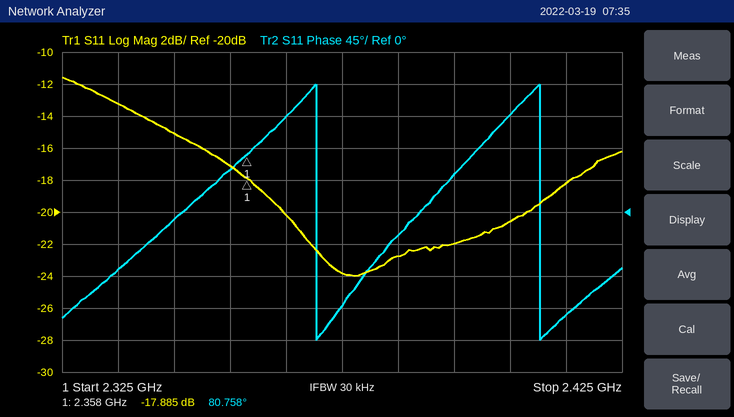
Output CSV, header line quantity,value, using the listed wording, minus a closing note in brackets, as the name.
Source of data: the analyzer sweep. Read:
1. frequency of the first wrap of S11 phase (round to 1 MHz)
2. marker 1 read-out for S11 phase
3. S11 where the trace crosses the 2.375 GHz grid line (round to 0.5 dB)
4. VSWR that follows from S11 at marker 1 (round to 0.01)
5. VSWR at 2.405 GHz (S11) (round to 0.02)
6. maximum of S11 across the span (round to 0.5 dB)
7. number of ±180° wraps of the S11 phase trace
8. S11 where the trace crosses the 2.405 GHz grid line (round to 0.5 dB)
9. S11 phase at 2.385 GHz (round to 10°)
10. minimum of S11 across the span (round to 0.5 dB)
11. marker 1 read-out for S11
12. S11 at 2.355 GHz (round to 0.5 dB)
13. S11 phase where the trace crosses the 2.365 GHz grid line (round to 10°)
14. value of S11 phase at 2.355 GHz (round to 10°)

quantity,value
frequency of the first wrap of S11 phase,2.370 GHz
marker 1 read-out for S11 phase,80.758°
S11 where the trace crosses the 2.375 GHz grid line,-24.0 dB
VSWR that follows from S11 at marker 1,1.29
VSWR at 2.405 GHz (S11),1.20
maximum of S11 across the span,-11.5 dB
number of ±180° wraps of the S11 phase trace,2
S11 where the trace crosses the 2.405 GHz grid line,-20.5 dB
S11 phase at 2.385 GHz,-30°
minimum of S11 across the span,-24.0 dB
marker 1 read-out for S11,-17.885 dB
S11 at 2.355 GHz,-17.0 dB
S11 phase where the trace crosses the 2.365 GHz grid line,130°
value of S11 phase at 2.355 GHz,60°
